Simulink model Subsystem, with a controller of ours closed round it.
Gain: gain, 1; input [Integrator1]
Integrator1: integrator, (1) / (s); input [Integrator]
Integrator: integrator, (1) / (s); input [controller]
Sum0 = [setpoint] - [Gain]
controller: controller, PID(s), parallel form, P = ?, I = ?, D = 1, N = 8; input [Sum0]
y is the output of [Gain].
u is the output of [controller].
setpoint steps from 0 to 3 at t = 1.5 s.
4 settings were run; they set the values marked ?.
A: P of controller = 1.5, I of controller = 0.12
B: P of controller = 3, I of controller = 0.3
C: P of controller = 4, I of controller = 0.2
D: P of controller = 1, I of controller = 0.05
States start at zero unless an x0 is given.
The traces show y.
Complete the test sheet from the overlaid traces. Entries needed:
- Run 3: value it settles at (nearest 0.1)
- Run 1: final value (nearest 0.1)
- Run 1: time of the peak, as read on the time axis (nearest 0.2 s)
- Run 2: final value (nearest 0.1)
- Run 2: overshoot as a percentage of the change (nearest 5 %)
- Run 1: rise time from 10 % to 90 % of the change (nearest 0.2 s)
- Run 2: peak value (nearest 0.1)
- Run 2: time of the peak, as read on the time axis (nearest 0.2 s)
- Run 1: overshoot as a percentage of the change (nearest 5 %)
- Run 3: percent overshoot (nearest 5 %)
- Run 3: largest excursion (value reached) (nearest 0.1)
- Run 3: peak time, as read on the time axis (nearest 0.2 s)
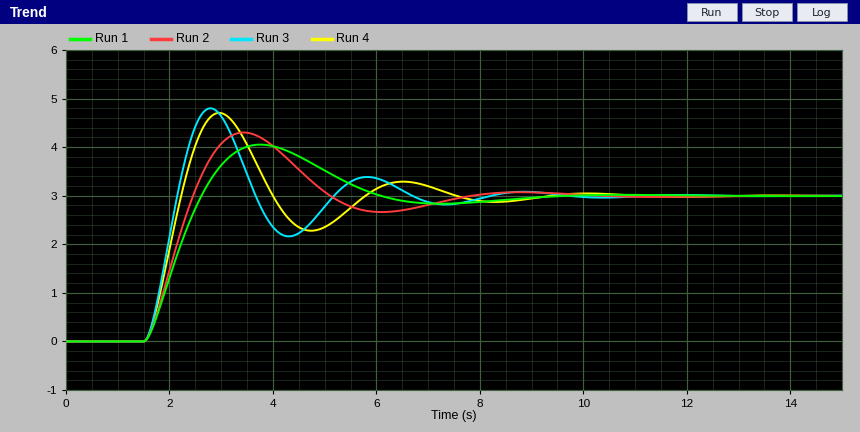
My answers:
3.0
3.0
3.8 s
3.0
45 %
0.8 s
4.3
3.4 s
35 %
60 %
4.8
2.8 s
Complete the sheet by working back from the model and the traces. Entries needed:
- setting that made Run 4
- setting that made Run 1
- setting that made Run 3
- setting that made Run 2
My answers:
B
D
C
A
